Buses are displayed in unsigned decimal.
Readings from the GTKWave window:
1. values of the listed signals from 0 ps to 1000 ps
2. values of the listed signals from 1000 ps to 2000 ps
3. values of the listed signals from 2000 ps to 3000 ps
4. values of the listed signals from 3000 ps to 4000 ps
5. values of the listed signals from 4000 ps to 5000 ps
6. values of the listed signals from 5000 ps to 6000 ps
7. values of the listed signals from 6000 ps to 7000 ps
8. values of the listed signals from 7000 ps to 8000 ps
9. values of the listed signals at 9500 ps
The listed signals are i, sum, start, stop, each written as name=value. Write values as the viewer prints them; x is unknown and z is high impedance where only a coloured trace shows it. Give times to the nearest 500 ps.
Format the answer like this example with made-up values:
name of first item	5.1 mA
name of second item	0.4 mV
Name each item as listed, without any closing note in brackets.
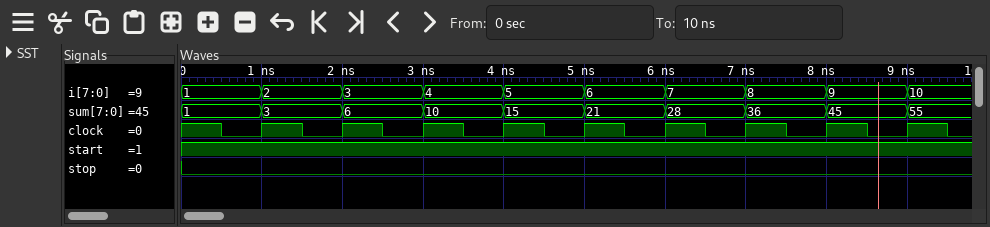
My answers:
values of the listed signals from 0 ps to 1000 ps	i=1, sum=1, start=1, stop=0
values of the listed signals from 1000 ps to 2000 ps	i=2, sum=3, start=1, stop=0
values of the listed signals from 2000 ps to 3000 ps	i=3, sum=6, start=1, stop=0
values of the listed signals from 3000 ps to 4000 ps	i=4, sum=10, start=1, stop=0
values of the listed signals from 4000 ps to 5000 ps	i=5, sum=15, start=1, stop=0
values of the listed signals from 5000 ps to 6000 ps	i=6, sum=21, start=1, stop=0
values of the listed signals from 6000 ps to 7000 ps	i=7, sum=28, start=1, stop=0
values of the listed signals from 7000 ps to 8000 ps	i=8, sum=36, start=1, stop=0
values of the listed signals at 9500 ps	i=10, sum=55, start=1, stop=0
